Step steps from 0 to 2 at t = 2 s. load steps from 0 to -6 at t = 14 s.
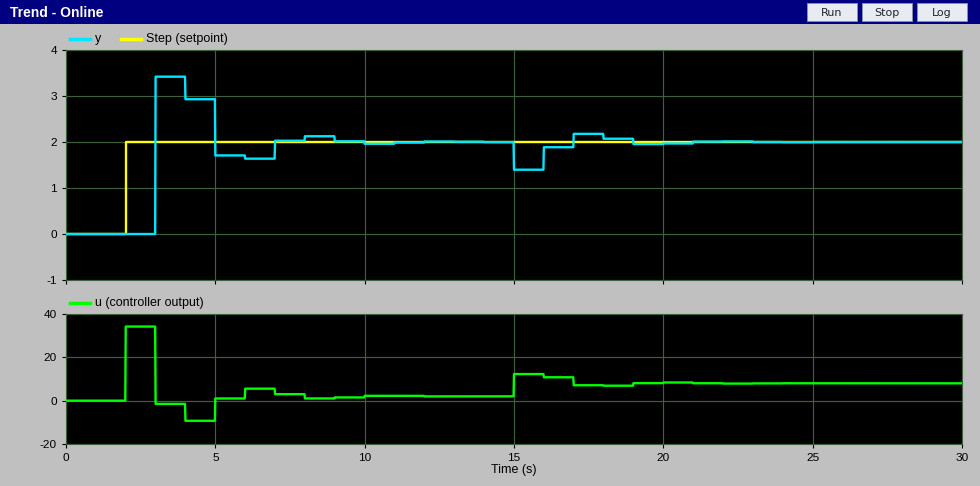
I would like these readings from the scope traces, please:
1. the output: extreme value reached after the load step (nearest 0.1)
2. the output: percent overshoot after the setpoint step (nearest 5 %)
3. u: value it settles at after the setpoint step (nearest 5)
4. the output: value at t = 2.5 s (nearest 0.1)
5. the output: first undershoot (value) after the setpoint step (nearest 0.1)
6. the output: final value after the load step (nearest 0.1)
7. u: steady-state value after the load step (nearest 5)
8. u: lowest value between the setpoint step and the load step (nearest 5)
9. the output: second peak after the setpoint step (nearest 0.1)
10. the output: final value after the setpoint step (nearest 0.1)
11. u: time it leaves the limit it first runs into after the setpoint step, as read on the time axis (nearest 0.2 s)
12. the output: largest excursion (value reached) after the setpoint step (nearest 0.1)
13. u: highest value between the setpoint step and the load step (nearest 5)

1.4
70 %
0
0.0
1.6
2.0
10
-10
2.1
2.0
3.0 s
3.4
35
